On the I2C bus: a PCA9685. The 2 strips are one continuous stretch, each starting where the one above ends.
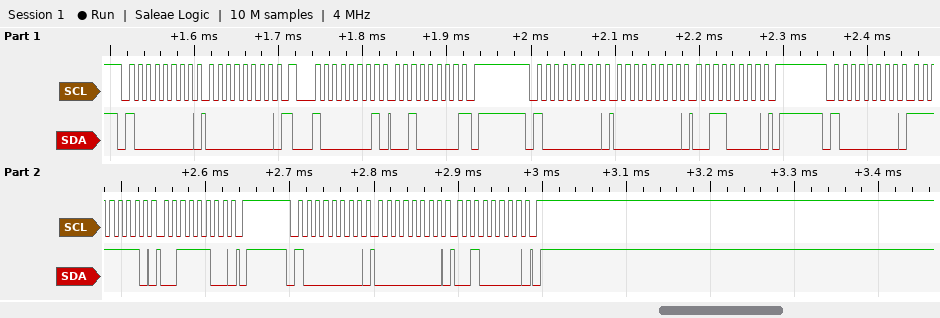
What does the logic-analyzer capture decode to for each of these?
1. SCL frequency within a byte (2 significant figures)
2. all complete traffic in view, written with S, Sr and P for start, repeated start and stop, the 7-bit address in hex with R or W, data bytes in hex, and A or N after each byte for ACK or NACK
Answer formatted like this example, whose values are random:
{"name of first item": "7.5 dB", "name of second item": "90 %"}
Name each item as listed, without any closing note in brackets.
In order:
{"SCL frequency within a byte": "100 kHz", "all complete traffic in view, written with S, Sr and P for start, repeated start and stop, the 7-bit address in hex with R or W, data bytes in hex, and A or N after each byte for ACK or NACK": "S 40W A 00 A Sr 40R A 20 N P S 40W A 00 A 30 A P S 40W A FE A 3C A P S 40W A 00 A 20 A P"}
